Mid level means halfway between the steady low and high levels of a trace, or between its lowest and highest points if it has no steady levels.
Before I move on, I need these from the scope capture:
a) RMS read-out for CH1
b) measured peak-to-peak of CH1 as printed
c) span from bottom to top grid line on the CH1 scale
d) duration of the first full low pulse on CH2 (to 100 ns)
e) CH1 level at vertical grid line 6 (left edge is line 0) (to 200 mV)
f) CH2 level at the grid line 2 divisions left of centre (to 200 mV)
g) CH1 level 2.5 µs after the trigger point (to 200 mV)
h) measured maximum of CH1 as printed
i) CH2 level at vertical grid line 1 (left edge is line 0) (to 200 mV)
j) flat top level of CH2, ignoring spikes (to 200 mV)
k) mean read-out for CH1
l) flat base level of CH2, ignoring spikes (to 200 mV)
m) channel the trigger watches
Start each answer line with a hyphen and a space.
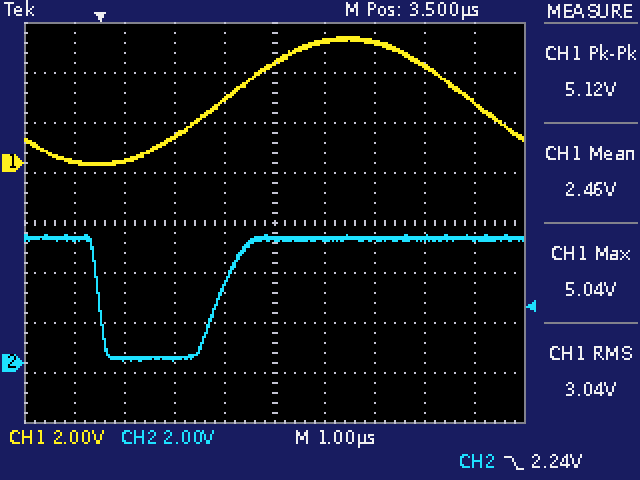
- 3.04 V
- 5.12 V
- 16 V
- 2.4 µs
- 4.8 V
- 200 mV
- 2.6 V
- 5.04 V
- 5.0 V
- 5.0 V
- 2.46 V
- 200 mV
- CH2
